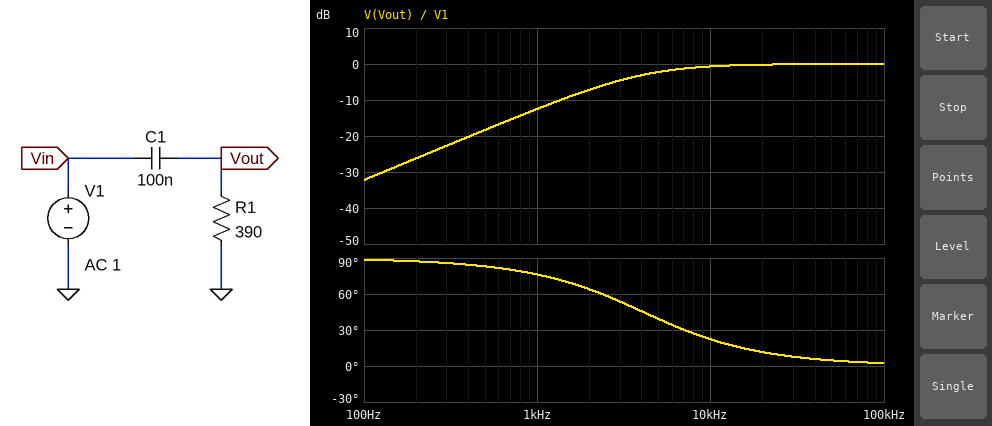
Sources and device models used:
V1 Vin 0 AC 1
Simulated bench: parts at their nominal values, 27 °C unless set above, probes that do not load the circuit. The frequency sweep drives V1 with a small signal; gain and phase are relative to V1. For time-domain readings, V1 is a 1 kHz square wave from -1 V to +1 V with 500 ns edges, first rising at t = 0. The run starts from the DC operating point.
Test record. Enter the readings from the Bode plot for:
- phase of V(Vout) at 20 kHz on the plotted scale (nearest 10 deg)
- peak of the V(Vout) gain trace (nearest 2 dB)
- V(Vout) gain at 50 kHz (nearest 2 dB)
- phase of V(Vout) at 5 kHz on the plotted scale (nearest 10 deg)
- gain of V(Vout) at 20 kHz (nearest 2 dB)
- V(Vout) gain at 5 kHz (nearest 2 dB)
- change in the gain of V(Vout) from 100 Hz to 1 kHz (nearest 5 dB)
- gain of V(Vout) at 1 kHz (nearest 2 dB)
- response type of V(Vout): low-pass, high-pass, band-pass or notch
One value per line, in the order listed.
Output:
10 deg
0 dB
0 dB
40 deg
0 dB
-2 dB
20 dB
-12 dB
high-pass
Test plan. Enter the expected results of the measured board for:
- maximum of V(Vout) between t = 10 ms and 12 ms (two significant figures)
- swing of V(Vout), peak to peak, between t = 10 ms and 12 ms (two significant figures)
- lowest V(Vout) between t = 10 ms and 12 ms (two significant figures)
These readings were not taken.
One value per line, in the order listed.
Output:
2.0 V
4.0 V
-2.0 V
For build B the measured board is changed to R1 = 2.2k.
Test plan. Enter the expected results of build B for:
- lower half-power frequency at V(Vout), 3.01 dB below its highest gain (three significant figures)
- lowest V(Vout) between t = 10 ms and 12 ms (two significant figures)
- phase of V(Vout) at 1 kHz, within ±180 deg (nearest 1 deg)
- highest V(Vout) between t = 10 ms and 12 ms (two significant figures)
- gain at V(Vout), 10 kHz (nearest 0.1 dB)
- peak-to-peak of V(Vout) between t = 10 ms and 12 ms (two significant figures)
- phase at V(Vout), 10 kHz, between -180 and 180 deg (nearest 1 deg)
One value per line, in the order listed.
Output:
723 Hz
-1.8 V
36 deg
1.8 V
0 dB
3.6 V
4 deg
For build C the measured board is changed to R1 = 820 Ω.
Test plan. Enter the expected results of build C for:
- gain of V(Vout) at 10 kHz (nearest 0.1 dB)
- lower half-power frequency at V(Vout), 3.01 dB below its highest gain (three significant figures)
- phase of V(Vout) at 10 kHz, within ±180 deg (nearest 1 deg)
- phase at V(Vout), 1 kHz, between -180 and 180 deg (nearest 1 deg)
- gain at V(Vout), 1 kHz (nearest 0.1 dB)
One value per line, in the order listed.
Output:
-0.2 dB
1.94 kHz
11 deg
63 deg
-6.8 dB
